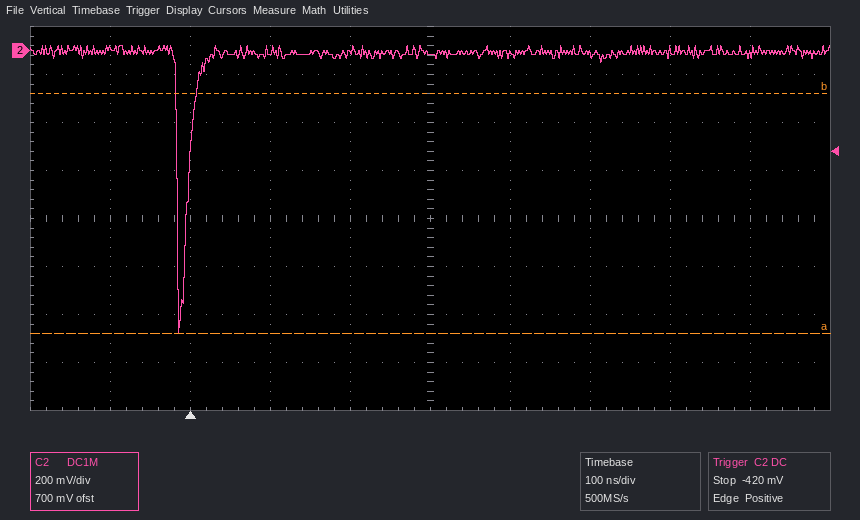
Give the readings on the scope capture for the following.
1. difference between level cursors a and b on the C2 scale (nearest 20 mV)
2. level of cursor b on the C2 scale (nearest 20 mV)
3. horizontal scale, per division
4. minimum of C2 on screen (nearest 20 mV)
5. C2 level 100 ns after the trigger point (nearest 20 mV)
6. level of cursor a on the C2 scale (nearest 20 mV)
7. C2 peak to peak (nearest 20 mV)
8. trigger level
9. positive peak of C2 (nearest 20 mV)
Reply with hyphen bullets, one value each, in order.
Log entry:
- 1.00 V
- -180 mV
- 100 ns
- -1.18 V
- 0 mV
- -1.18 V
- 1.20 V
- -420 mV
- 20 mV
